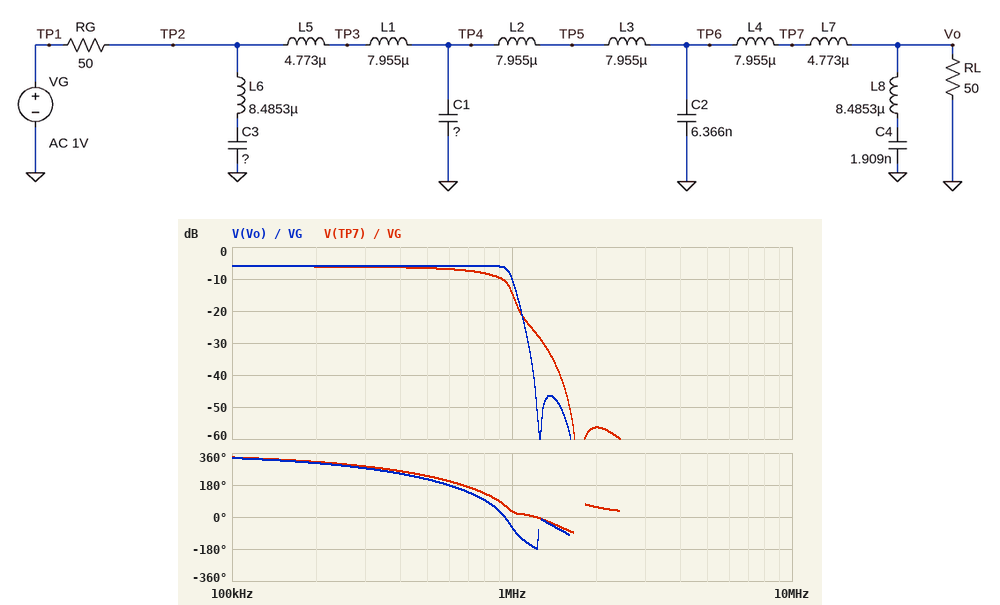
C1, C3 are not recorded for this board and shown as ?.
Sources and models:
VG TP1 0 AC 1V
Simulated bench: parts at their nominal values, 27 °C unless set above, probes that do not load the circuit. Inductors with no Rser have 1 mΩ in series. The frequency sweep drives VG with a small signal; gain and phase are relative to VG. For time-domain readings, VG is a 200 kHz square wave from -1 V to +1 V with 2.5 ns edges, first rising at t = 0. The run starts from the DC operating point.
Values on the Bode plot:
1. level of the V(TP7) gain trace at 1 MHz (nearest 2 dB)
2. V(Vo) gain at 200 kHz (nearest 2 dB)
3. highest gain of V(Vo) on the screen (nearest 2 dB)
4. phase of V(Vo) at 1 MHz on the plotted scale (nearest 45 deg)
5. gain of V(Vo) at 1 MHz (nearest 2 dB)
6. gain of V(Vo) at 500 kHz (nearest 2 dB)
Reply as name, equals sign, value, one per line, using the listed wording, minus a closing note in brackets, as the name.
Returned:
level of the V(TP7) gain trace at 1 MHz = -14 dB
V(Vo) gain at 200 kHz = -6 dB
highest gain of V(Vo) on the screen = -6 dB
phase of V(Vo) at 1 MHz on the plotted scale = -45 deg
gain of V(Vo) at 1 MHz = -10 dB
gain of V(Vo) at 500 kHz = -6 dB
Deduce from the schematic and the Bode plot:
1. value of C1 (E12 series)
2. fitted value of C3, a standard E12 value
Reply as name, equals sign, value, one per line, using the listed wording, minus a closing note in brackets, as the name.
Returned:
value of C1 = 5.6 nF
fitted value of C3, a standard E12 value = 1 nF
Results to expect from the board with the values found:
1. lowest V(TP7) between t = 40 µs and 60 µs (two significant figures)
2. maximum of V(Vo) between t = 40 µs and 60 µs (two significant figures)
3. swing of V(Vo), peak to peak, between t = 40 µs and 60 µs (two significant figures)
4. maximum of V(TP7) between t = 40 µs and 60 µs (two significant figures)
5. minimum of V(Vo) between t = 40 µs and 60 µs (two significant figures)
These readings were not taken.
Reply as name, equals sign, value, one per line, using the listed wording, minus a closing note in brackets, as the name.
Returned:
lowest V(TP7) between t = 40 µs and 60 µs = -630 mV
maximum of V(Vo) between t = 40 µs and 60 µs = 710 mV
swing of V(Vo), peak to peak, between t = 40 µs and 60 µs = 1.4 V
maximum of V(TP7) between t = 40 µs and 60 µs = 630 mV
minimum of V(Vo) between t = 40 µs and 60 µs = -710 mV
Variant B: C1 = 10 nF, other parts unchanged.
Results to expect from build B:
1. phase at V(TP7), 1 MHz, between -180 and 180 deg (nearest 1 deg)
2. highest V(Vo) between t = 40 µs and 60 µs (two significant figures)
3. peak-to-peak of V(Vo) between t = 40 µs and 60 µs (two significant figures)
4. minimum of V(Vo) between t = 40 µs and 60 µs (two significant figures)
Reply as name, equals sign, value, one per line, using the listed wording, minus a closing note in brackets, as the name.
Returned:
phase at V(TP7), 1 MHz, between -180 and 180 deg = -7 deg
highest V(Vo) between t = 40 µs and 60 µs = 650 mV
peak-to-peak of V(Vo) between t = 40 µs and 60 µs = 1.3 V
minimum of V(Vo) between t = 40 µs and 60 µs = -650 mV
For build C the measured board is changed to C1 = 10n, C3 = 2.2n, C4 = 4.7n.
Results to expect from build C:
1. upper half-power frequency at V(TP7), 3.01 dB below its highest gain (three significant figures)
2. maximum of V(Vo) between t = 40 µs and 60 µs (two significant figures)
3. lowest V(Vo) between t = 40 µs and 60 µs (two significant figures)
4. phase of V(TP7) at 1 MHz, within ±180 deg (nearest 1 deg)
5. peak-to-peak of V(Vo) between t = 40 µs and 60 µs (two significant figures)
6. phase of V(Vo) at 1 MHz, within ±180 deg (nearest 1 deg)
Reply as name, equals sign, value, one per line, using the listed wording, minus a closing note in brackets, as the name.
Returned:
upper half-power frequency at V(TP7), 3.01 dB below its highest gain = 848 kHz
maximum of V(Vo) between t = 40 µs and 60 µs = 640 mV
lowest V(Vo) between t = 40 µs and 60 µs = -640 mV
phase of V(TP7) at 1 MHz, within ±180 deg = -62 deg
peak-to-peak of V(Vo) between t = 40 µs and 60 µs = 1.3 V
phase of V(Vo) at 1 MHz, within ±180 deg = -76 deg
